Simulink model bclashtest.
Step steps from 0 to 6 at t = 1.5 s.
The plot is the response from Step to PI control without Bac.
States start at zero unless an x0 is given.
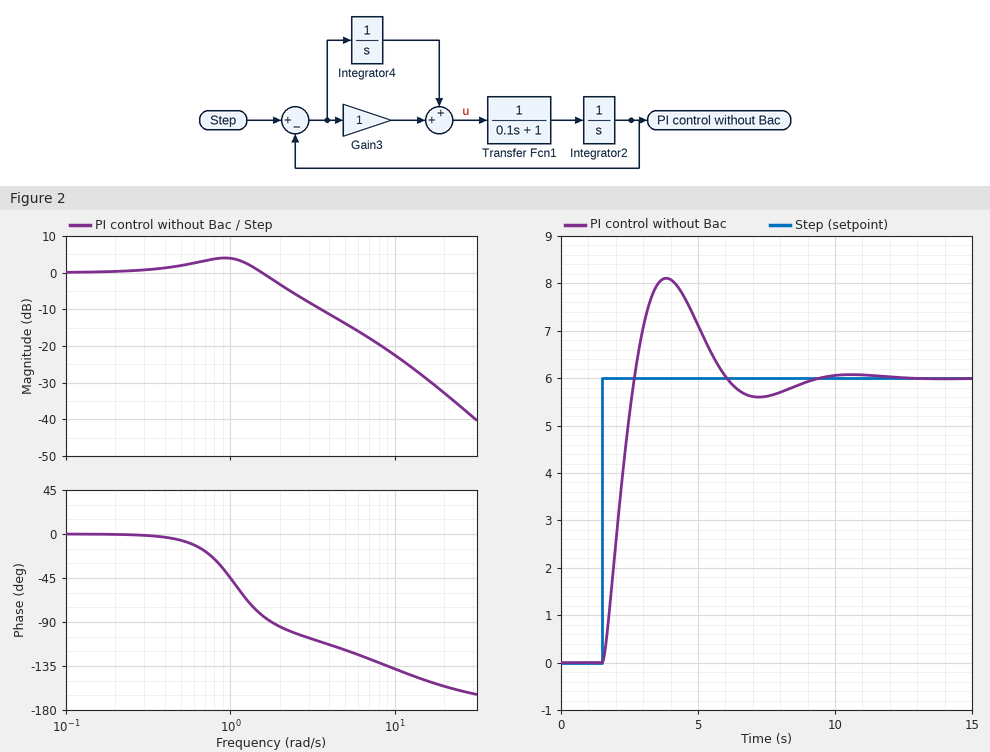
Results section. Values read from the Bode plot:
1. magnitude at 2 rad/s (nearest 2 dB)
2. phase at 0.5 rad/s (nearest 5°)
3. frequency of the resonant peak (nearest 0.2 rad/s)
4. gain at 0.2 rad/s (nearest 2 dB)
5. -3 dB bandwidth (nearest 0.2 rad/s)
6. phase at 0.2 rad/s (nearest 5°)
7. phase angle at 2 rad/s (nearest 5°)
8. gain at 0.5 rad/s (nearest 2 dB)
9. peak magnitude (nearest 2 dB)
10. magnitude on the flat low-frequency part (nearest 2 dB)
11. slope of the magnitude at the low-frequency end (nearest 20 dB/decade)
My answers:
-4 dB
-5°
1.0 rad/s
0 dB
2.0 rad/s
0°
-95°
2 dB
4 dB
0 dB
0 dB/decade
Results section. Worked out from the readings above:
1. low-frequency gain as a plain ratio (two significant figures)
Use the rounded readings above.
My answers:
1.0
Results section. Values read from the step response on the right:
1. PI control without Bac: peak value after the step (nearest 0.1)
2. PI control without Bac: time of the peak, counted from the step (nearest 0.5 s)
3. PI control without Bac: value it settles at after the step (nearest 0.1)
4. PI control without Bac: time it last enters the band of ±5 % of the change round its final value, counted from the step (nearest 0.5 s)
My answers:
8.1
2.5 s
6.0
6.5 s
